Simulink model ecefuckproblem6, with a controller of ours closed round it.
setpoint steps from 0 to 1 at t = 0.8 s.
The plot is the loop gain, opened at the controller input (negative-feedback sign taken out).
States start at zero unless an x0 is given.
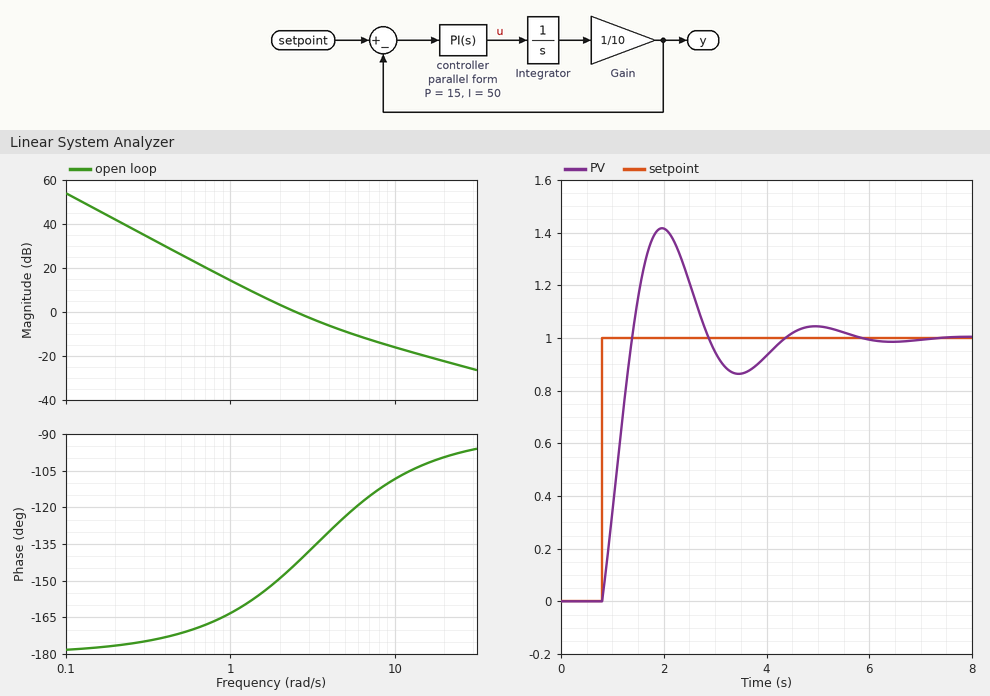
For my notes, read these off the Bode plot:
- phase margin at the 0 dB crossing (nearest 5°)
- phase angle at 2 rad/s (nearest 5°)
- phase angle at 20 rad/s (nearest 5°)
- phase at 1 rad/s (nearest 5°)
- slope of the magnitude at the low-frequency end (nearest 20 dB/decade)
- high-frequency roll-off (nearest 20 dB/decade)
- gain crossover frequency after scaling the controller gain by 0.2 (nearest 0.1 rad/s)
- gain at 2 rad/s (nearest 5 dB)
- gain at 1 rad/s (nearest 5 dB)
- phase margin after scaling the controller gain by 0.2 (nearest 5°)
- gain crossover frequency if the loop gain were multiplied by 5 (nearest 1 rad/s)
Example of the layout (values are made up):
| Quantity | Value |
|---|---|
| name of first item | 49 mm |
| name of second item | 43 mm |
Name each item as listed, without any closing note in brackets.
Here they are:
| Quantity | Value |
|---|---|
| phase margin at the 0 dB crossing | 35° |
| phase angle at 2 rad/s | -150° |
| phase angle at 20 rad/s | -100° |
| phase at 1 rad/s | -165° |
| slope of the magnitude at the low-frequency end | -40 dB/decade |
| high-frequency roll-off | -20 dB/decade |
| gain crossover frequency after scaling the controller gain by 0.2 | 1.0 rad/s |
| gain at 2 rad/s | 5 dB |
| gain at 1 rad/s | 15 dB |
| phase margin after scaling the controller gain by 0.2 | 15° |
| gain crossover frequency if the loop gain were multiplied by 5 | 8 rad/s |
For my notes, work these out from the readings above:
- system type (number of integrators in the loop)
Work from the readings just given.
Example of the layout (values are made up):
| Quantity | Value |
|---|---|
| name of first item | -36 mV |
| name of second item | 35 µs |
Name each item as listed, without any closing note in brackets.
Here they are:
| Quantity | Value |
|---|---|
| system type | 2 |
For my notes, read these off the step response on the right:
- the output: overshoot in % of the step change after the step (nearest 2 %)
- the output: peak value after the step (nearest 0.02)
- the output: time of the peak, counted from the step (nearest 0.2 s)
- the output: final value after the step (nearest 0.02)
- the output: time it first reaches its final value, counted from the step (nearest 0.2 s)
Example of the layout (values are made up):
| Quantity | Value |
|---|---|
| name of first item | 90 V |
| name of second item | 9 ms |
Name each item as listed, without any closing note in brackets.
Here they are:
| Quantity | Value |
|---|---|
| the output: overshoot in % of the step change after the step | 42 % |
| the output: peak value after the step | 1.42 |
| the output: time of the peak, counted from the step | 1.2 s |
| the output: final value after the step | 1.00 |
| the output: time it first reaches its final value, counted from the step | 0.6 s |
